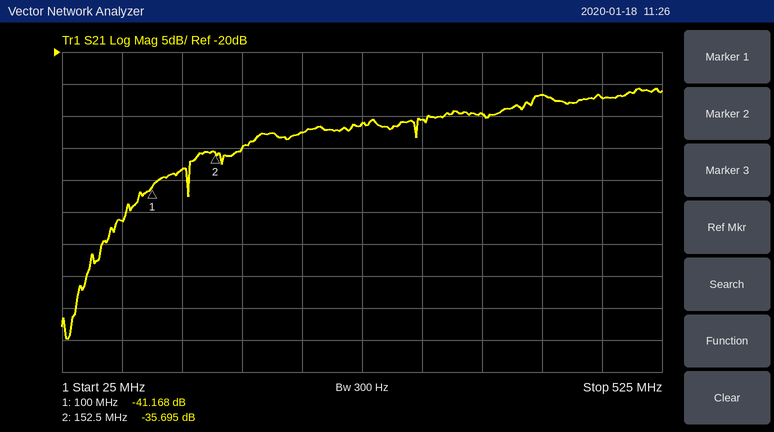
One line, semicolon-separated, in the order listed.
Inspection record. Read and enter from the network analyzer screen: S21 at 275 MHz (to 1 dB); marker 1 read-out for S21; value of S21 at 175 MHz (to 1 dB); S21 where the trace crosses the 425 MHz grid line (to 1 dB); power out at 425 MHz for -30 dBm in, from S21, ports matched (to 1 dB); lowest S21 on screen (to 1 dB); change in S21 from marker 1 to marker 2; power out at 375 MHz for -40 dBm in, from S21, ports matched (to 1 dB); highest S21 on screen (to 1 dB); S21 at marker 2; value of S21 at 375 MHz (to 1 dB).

-31 dB; -41.168 dB; -35 dB; -27 dB; -57 dBm; -65 dB; 5.473 dB; -70 dBm; -26 dB; -35.695 dB; -30 dB
